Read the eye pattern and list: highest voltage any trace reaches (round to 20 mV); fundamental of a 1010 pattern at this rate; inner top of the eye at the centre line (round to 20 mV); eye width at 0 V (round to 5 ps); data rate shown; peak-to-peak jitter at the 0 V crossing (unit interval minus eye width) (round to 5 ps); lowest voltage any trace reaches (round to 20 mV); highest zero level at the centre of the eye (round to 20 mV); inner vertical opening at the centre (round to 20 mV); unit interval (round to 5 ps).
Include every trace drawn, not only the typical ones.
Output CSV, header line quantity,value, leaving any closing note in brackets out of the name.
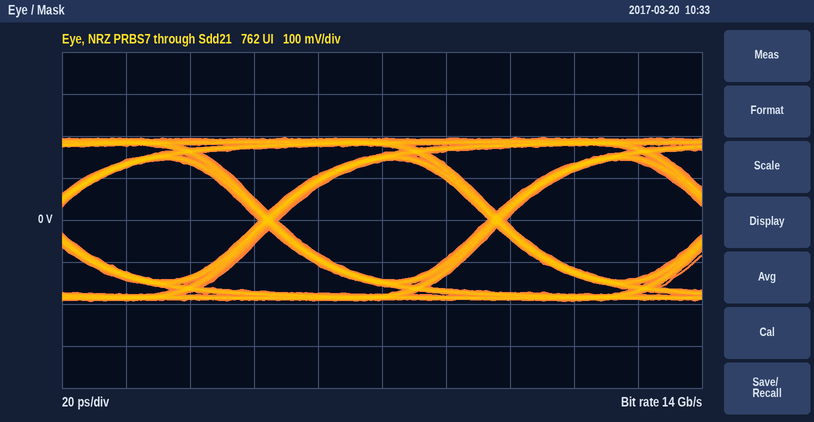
quantity,value
highest voltage any trace reaches,200 mV
fundamental of a 1010 pattern at this rate,7 GHz
inner top of the eye at the centre line,140 mV
eye width at 0 V,65 ps
data rate shown,14 Gb/s
peak-to-peak jitter at the 0 V crossing (unit interval minus eye width),5 ps
lowest voltage any trace reaches,-200 mV
highest zero level at the centre of the eye,-140 mV
inner vertical opening at the centre,280 mV
unit interval,70 ps
